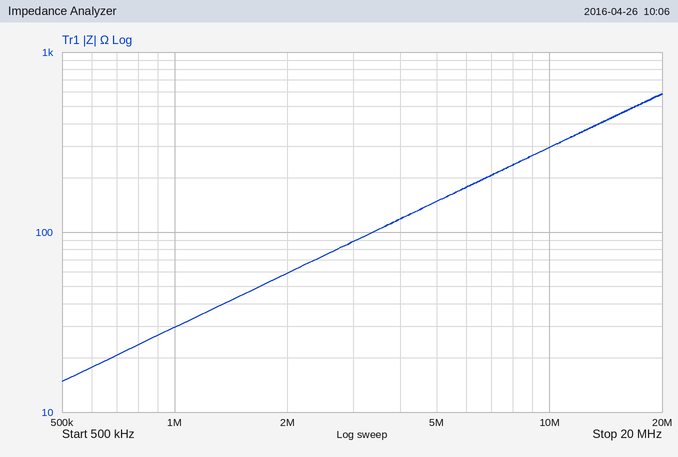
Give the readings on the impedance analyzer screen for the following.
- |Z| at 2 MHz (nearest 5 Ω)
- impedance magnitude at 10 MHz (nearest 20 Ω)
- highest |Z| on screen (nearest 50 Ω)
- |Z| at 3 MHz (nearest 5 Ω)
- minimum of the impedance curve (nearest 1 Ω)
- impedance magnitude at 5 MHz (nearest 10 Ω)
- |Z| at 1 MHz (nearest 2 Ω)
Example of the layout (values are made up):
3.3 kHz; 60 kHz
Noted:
60 Ω; 300 Ω; 600 Ω; 90 Ω; 15 Ω; 150 Ω; 30 Ω
